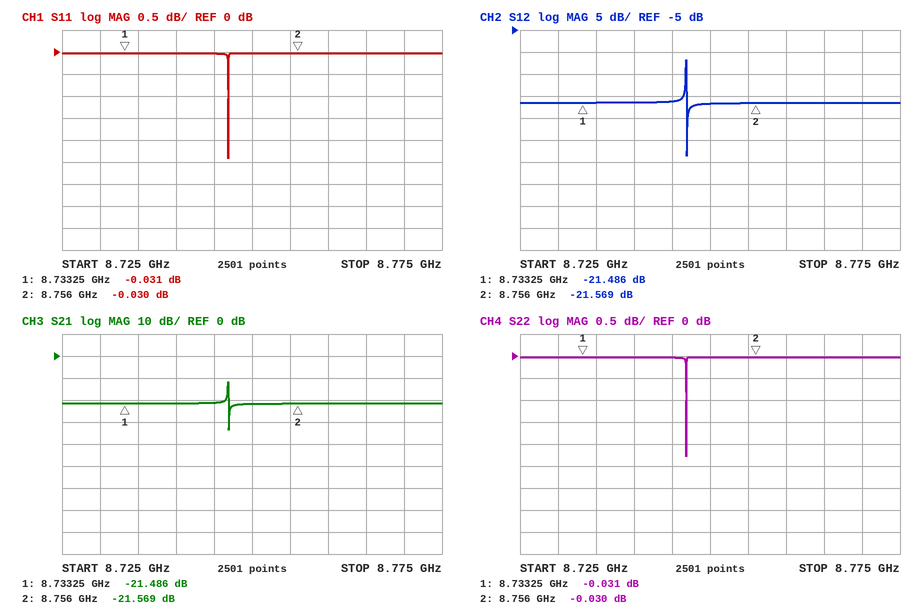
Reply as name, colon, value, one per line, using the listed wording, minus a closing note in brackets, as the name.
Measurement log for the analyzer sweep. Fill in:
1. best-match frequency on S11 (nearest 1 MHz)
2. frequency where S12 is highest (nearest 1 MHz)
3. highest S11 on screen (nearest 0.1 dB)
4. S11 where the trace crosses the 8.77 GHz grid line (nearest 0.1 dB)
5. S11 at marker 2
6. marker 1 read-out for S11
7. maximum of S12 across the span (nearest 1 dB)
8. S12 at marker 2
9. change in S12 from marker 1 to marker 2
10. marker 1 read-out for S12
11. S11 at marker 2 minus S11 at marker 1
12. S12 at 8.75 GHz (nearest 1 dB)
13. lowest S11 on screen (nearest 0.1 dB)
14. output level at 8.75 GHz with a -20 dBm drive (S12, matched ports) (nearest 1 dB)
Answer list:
best-match frequency on S11: 8.747 GHz
frequency where S12 is highest: 8.747 GHz
highest S11 on screen: 0.0 dB
S11 where the trace crosses the 8.77 GHz grid line: 0.0 dB
S11 at marker 2: -0.030 dB
marker 1 read-out for S11: -0.031 dB
maximum of S12 across the span: -12 dB
S12 at marker 2: -21.569 dB
change in S12 from marker 1 to marker 2: -0.083 dB
marker 1 read-out for S12: -21.486 dB
S11 at marker 2 minus S11 at marker 1: 0.001 dB
S12 at 8.75 GHz: -22 dB
lowest S11 on screen: -2.4 dB
output level at 8.75 GHz with a -20 dBm drive (S12, matched ports): -42 dBm
